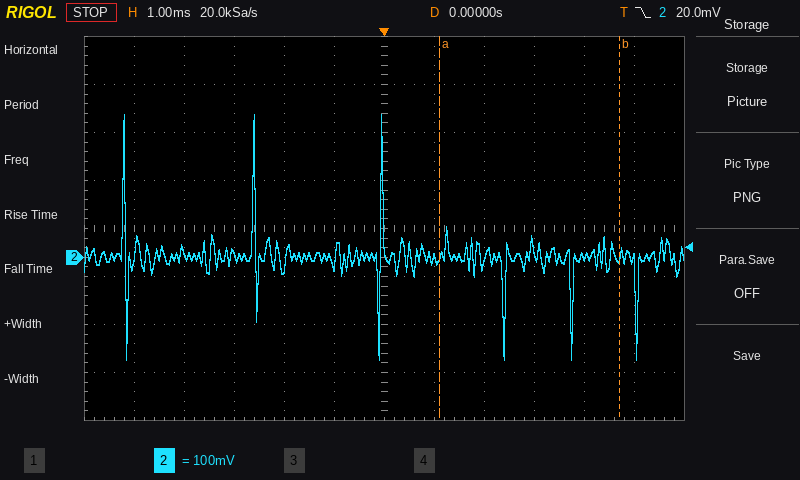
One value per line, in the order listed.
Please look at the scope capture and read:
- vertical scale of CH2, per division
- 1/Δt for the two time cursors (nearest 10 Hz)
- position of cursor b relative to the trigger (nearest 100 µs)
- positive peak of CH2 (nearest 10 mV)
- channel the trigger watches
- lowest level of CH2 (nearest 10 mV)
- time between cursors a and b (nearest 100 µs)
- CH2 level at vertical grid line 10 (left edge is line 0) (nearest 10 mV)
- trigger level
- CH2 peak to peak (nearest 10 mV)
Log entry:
100 mV
280 Hz
+4.7 ms
300 mV
CH2
-210 mV
3.6 ms
0 mV
20.0 mV
510 mV
